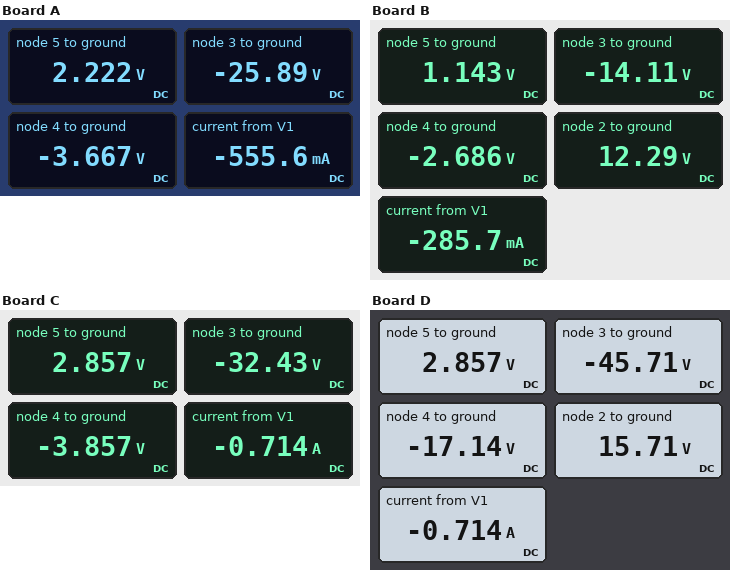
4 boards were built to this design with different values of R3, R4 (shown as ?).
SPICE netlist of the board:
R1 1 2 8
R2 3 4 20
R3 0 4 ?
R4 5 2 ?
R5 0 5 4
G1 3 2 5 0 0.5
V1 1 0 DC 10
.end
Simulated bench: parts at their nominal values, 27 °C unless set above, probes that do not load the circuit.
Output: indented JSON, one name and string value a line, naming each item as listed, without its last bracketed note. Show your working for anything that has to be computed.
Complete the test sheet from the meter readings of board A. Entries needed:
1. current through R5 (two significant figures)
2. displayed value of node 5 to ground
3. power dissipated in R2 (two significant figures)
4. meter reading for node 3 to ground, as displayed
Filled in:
{
  "current through R5": "(2.222 V) / 4 Ω = 560 mA",
  "displayed value of node 5 to ground": "2.222 V",
  "power dissipated in R2": "(-3.667 V - (-25.89 V))^2 / 20 Ω = 25 W",
  "meter reading for node 3 to ground, as displayed": "-25.89 V"
}
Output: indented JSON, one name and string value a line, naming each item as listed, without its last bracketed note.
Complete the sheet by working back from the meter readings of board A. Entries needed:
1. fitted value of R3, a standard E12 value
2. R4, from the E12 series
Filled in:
{
  "fitted value of R3, a standard E12 value": "3.3 Ω",
  "R4, from the E12 series": "22 Ω"
}
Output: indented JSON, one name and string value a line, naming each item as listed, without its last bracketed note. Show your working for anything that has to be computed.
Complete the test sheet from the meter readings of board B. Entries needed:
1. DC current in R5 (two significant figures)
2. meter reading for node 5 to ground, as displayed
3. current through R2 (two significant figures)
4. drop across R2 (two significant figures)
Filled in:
{
  "DC current in R5": "(1.143 V) / 4 Ω = 290 mA",
  "meter reading for node 5 to ground, as displayed": "1.143 V",
  "current through R2": "(-2.686 V - (-14.11 V)) / 20 Ω = 570 mA",
  "drop across R2": "-2.686 V - (-14.11 V) = 11 V"
}
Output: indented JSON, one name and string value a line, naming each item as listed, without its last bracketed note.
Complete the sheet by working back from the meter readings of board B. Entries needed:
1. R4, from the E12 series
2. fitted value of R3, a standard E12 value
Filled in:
{
  "R4, from the E12 series": "39 Ω",
  "fitted value of R3, a standard E12 value": "4.7 Ω"
}
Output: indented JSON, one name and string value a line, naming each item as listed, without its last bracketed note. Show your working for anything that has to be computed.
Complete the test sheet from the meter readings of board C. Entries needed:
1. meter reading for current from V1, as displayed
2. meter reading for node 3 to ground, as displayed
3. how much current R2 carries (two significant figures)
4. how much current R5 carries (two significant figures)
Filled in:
{
  "meter reading for current from V1, as displayed": "-0.714 A",
  "meter reading for node 3 to ground, as displayed": "-32.43 V",
  "how much current R2 carries": "(-3.857 V - (-32.43 V)) / 20 Ω = 1.4 A",
  "how much current R5 carries": "(2.857 V) / 4 Ω = 710 mA"
}
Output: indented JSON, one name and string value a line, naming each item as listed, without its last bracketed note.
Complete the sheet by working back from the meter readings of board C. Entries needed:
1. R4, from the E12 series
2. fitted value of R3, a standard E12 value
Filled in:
{
  "R4, from the E12 series": "18 Ω",
  "fitted value of R3, a standard E12 value": "2.7 Ω"
}
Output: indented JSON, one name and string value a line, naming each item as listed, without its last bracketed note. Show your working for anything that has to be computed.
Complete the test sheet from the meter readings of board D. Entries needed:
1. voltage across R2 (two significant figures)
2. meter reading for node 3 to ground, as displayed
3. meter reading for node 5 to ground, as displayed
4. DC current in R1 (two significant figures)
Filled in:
{
  "voltage across R2": "-17.14 V - (-45.71 V) = 29 V",
  "meter reading for node 3 to ground, as displayed": "-45.71 V",
  "meter reading for node 5 to ground, as displayed": "2.857 V",
  "DC current in R1": "(15.71 V - 10 V) / 8 Ω = 710 mA"
}
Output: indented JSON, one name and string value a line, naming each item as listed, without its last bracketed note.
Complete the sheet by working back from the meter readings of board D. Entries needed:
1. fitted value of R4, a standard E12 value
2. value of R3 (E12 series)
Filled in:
{
  "fitted value of R4, a standard E12 value": "18 Ω",
  "value of R3": "12 Ω"
}
